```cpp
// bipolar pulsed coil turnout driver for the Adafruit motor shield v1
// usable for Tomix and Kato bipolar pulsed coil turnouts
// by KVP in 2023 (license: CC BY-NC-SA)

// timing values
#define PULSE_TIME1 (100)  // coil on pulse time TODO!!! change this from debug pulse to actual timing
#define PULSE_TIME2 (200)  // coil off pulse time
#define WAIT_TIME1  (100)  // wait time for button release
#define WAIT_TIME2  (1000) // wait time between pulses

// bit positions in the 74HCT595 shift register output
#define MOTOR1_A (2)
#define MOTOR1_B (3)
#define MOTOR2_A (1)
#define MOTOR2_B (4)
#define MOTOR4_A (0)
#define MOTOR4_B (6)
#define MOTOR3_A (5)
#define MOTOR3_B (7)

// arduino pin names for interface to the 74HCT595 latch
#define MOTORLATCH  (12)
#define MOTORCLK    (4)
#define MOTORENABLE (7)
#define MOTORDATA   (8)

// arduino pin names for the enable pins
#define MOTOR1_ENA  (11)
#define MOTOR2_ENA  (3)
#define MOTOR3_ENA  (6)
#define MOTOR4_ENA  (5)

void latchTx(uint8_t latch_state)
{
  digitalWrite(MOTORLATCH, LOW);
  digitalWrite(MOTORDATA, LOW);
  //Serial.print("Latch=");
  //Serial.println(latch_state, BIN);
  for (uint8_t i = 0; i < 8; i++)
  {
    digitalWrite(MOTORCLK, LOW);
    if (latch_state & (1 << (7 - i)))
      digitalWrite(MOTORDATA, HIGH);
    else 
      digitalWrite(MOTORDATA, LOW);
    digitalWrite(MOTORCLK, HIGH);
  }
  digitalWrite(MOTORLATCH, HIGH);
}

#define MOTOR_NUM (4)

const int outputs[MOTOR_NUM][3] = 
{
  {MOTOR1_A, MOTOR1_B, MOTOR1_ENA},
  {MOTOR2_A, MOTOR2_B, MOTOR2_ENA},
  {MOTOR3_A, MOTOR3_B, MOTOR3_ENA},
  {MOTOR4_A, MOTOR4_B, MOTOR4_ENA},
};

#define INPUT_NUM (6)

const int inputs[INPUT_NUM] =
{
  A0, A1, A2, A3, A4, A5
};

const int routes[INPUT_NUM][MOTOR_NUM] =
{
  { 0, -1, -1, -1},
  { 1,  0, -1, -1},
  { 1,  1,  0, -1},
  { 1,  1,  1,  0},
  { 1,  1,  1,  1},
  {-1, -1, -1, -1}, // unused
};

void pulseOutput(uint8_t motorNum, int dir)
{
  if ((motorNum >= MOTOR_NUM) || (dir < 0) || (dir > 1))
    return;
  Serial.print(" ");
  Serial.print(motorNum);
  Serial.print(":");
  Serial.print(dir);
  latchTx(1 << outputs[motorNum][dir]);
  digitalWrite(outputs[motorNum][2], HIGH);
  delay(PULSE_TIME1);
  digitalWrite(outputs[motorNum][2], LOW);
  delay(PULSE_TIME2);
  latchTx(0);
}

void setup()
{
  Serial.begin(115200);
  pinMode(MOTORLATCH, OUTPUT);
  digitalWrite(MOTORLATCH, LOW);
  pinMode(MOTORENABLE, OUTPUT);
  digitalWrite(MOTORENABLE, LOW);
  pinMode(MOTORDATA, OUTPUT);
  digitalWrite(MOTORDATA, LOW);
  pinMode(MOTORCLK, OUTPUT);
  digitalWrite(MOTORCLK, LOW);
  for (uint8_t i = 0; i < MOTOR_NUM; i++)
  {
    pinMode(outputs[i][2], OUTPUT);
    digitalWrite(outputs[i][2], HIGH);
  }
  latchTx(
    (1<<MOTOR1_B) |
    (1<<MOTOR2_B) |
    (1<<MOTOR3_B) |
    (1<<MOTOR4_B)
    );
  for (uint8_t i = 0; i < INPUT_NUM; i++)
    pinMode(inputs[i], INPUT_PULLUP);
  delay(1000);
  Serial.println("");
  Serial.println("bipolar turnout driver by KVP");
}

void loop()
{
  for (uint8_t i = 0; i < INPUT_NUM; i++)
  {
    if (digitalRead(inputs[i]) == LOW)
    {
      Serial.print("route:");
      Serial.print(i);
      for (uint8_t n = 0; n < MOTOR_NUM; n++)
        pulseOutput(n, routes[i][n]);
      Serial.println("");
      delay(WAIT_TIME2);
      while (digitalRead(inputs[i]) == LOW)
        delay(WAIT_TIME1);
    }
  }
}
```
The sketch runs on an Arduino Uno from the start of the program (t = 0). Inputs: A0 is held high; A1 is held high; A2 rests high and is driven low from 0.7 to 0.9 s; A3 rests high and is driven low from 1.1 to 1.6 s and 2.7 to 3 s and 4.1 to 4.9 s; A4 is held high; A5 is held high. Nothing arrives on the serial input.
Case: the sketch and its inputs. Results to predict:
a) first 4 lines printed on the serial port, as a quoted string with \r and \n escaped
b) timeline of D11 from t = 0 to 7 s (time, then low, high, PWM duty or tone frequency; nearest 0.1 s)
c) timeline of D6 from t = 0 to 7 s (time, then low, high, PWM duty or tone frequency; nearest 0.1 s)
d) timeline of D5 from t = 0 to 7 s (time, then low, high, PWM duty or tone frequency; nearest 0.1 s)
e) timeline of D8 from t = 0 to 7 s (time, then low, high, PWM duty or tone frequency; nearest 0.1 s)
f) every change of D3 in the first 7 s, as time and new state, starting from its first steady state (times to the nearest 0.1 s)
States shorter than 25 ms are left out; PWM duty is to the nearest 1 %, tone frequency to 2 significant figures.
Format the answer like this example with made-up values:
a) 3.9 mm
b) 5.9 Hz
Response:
a) "\r\nbipolar turnout driver by KVP\r\nroute:3 0:1 1:1 2:1 3:0\r\nroute:3 0:1 1:1 2:1 3:0\r\n"
b) 0 s high; 1.2 s low; 4.1 s high; 4.2 s low
c) 0 s high; 1.8 s low; 4.7 s high; 4.8 s low
d) 0 s high; 2.1 s low; 5 s high; 5.1 s low
e) 0 s low; 2 s high; 2.3 s low; 5 s high; 5.3 s low
f) 0 s high; 1.5 s low; 4.4 s high; 4.5 s low
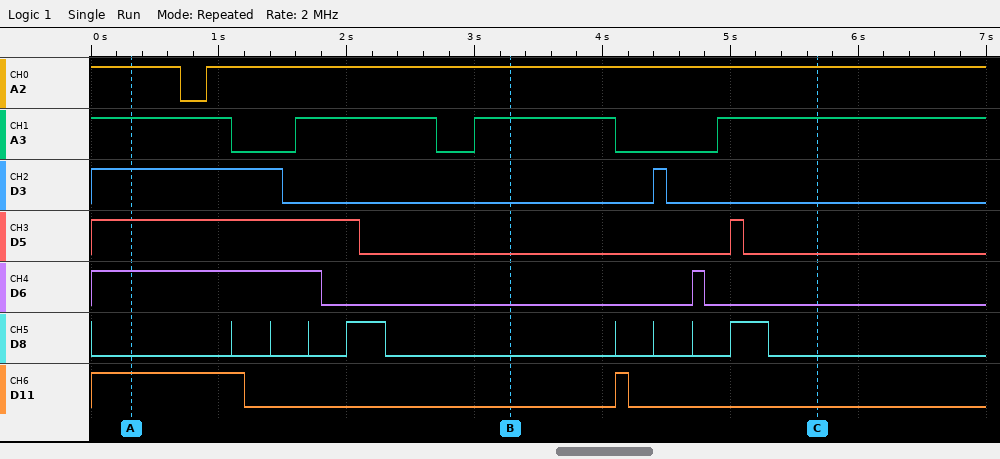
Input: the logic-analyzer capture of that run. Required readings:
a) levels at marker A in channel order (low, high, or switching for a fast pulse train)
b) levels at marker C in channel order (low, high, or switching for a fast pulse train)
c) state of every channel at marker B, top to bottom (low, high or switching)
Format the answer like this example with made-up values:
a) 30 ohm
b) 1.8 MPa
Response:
a) A2 high, A3 high, D3 high, D5 high, D6 high, D8 low, D11 high
b) A2 high, A3 high, D3 low, D5 low, D6 low, D8 low, D11 low
c) A2 high, A3 high, D3 low, D5 low, D6 low, D8 low, D11 low
